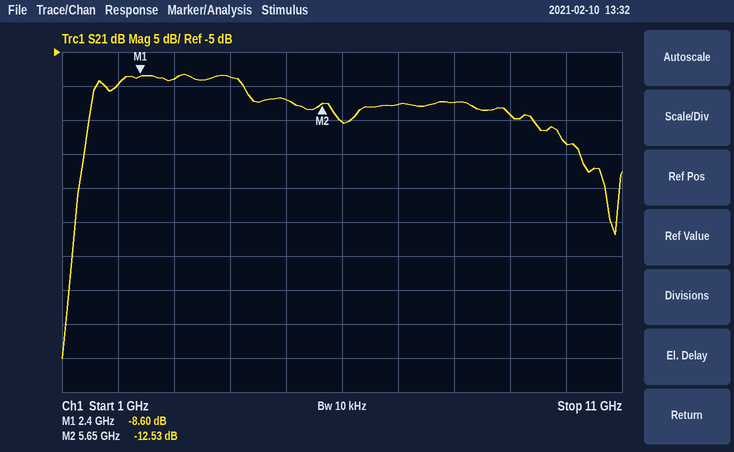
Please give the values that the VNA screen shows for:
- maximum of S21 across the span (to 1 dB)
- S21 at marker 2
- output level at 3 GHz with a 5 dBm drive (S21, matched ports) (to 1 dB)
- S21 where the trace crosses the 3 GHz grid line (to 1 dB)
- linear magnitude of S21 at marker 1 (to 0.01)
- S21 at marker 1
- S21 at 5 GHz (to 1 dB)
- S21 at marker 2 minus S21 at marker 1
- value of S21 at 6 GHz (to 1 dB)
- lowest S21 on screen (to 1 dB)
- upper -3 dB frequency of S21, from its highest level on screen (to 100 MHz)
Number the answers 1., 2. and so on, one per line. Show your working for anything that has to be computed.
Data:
1. -8 dB
2. -12.53 dB
3. 5 dBm + (-9 dB) = -4 dBm
4. -9 dB
5. 10^(-8.6/20) ≈ 0.37
6. -8.60 dB
7. -12 dB
8. -12.53 − (-8.6) = -3.93 dB
9. -15 dB
10. -50 dB
11. 4.3 GHz
